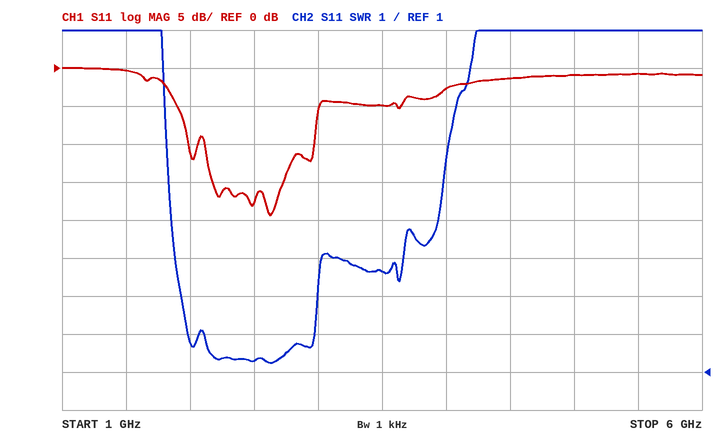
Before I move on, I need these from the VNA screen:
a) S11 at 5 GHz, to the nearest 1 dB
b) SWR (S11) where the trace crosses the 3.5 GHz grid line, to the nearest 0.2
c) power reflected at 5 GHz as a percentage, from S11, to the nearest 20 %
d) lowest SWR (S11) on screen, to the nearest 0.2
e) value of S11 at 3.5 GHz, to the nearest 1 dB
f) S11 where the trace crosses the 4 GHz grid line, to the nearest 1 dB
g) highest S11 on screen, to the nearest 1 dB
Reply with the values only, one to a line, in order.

-1 dB
3.6
80 %
1.2
-5 dB
-3 dB
0 dB
